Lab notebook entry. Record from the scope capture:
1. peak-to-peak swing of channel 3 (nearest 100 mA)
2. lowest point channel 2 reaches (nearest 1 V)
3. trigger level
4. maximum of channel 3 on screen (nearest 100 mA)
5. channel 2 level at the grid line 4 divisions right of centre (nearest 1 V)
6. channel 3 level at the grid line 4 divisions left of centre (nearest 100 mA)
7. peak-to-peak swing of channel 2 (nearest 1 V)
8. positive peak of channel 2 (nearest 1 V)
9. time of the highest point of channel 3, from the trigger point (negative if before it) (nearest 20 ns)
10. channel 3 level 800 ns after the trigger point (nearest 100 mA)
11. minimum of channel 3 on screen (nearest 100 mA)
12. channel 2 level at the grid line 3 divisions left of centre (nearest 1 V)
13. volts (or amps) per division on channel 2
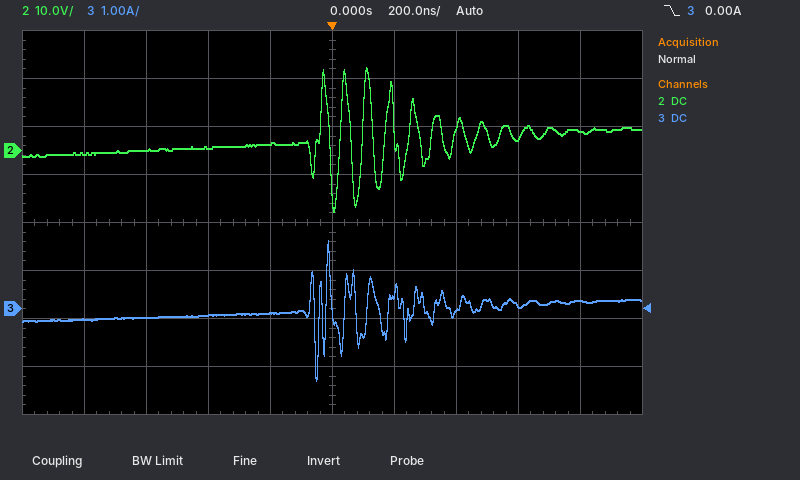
2.9 A
-13 V
0.00 A
1.4 A
4 V
-200 mA
30 V
17 V
-20 ns
200 mA
-1.5 A
0 V
10 V
